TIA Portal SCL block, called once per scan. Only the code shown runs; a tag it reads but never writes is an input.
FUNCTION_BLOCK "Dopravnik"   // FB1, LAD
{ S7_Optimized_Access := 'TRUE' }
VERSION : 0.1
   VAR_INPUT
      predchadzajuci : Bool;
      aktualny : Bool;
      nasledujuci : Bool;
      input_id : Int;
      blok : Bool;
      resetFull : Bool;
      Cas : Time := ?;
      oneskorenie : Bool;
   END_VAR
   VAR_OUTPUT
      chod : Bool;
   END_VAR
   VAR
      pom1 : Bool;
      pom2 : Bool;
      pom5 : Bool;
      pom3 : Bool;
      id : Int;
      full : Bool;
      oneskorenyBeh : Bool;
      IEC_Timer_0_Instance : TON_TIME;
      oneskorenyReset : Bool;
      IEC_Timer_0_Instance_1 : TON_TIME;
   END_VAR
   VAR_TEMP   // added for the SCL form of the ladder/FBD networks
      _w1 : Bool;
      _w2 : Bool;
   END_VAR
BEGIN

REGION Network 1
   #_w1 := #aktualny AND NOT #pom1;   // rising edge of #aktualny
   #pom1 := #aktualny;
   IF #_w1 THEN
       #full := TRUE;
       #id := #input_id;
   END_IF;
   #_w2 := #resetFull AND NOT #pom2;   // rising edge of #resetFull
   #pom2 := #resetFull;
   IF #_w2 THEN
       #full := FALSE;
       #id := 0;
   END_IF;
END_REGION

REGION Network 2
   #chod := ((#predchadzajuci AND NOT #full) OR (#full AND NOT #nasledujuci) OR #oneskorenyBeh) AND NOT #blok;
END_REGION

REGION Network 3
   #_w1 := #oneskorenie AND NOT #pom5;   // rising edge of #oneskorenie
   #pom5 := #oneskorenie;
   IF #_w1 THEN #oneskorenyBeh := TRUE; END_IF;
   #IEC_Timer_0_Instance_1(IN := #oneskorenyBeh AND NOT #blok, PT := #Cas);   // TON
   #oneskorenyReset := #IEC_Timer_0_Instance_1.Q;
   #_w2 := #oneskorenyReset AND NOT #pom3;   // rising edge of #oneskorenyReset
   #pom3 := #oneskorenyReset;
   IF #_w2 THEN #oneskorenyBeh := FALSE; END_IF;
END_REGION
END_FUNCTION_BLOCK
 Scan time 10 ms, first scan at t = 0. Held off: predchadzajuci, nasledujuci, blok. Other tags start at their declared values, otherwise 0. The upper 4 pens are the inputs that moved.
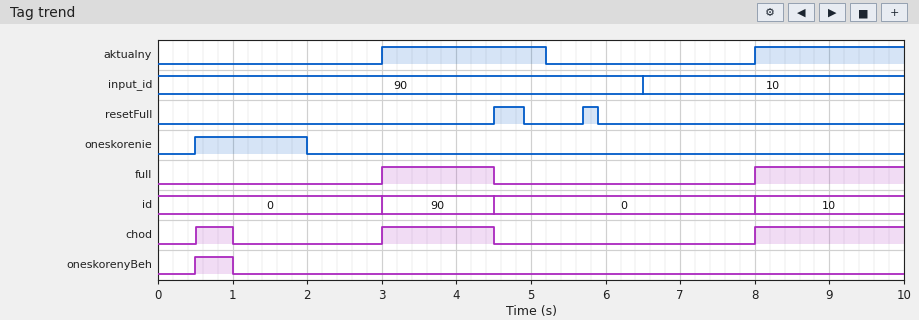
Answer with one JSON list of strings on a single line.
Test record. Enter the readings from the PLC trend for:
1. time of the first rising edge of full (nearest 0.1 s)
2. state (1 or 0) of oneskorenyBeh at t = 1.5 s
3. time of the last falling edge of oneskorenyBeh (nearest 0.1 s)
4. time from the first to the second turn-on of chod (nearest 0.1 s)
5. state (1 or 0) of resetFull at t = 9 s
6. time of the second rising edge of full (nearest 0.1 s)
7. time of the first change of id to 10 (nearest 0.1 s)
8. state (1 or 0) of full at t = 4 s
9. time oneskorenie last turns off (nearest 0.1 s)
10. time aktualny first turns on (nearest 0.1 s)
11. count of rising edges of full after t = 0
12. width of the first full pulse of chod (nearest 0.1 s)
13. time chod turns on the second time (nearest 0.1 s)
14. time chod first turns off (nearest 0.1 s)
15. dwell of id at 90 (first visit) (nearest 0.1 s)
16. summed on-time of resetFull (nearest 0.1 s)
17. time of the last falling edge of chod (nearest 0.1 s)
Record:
["3.0 s", "0", "1.0 s", "2.5 s", "0", "8.0 s", "8.0 s", "1", "2.0 s", "3.0 s", "2", "0.5 s", "3.0 s", "1.0 s", "1.5 s", "0.6 s", "4.5 s"]
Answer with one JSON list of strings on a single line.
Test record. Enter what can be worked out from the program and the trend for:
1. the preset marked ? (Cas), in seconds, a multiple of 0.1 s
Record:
["0.5 s"]
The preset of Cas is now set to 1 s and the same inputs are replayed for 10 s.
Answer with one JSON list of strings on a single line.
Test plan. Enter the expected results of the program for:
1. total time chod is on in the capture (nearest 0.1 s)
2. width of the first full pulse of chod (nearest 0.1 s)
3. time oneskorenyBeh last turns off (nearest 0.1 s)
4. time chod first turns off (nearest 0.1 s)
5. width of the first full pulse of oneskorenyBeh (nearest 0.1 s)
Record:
["4.5 s", "1.0 s", "1.5 s", "1.5 s", "1.0 s"]
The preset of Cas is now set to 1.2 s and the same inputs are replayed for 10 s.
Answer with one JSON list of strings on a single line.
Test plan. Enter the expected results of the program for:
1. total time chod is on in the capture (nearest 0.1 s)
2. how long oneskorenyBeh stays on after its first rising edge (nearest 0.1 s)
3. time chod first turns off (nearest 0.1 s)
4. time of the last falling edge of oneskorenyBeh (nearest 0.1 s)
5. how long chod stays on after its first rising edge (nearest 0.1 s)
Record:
["4.7 s", "1.2 s", "1.7 s", "1.7 s", "1.2 s"]
